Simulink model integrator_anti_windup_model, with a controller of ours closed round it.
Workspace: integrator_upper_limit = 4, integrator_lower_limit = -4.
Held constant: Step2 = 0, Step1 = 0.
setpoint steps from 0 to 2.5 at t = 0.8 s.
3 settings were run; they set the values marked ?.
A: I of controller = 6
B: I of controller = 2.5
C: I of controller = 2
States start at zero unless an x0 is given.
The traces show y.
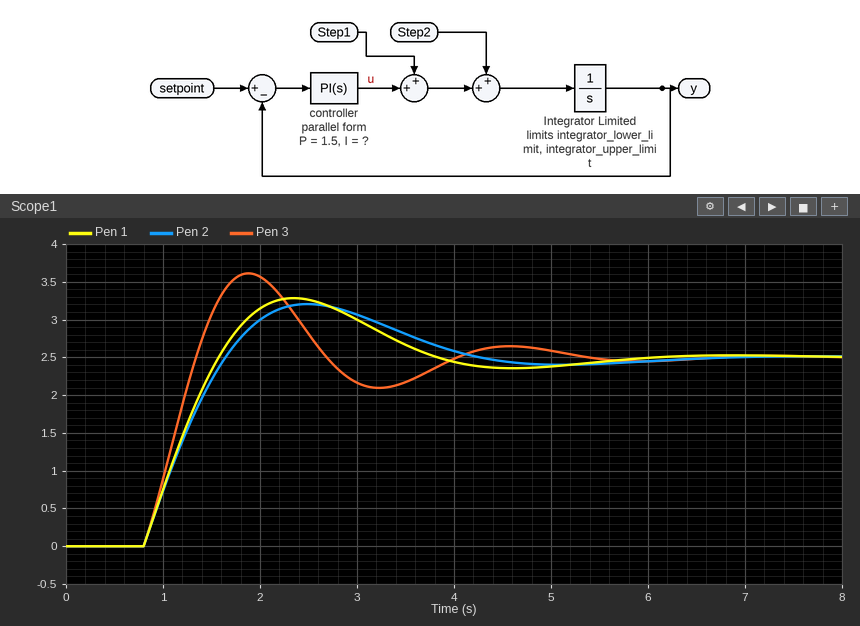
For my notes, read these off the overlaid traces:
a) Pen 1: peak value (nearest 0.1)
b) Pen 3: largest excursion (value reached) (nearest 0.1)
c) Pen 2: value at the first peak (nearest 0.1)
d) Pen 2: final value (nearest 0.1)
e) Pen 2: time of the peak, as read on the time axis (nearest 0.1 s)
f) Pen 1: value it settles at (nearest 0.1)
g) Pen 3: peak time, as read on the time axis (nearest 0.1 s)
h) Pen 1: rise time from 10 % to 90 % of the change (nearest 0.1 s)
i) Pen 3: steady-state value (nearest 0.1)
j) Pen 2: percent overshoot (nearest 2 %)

3.3
3.6
3.2
2.5
2.5 s
2.5
1.9 s
0.6 s
2.5
28 %
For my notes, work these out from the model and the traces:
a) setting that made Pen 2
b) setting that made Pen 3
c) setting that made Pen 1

C
A
B
